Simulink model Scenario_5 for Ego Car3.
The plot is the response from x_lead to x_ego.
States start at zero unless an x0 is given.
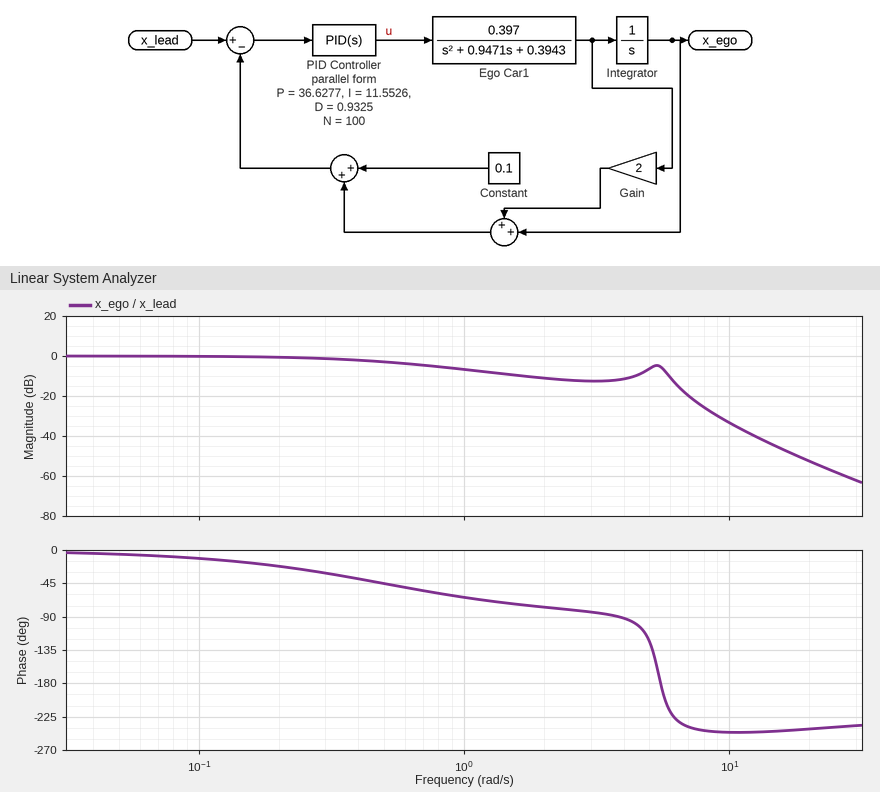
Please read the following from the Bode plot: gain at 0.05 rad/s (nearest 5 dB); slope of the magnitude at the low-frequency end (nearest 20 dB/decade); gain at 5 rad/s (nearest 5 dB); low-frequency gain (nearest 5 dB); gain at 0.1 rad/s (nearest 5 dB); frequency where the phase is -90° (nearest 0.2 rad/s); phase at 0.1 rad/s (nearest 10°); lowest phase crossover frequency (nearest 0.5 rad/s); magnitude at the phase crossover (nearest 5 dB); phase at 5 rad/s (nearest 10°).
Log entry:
0 dB
0 dB/decade
-5 dB
0 dB
0 dB
3.8 rad/s
-10°
5.5 rad/s
-5 dB
-120°
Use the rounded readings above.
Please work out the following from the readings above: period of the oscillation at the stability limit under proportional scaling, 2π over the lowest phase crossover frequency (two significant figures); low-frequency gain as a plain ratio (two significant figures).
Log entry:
1.1 s
1.0
